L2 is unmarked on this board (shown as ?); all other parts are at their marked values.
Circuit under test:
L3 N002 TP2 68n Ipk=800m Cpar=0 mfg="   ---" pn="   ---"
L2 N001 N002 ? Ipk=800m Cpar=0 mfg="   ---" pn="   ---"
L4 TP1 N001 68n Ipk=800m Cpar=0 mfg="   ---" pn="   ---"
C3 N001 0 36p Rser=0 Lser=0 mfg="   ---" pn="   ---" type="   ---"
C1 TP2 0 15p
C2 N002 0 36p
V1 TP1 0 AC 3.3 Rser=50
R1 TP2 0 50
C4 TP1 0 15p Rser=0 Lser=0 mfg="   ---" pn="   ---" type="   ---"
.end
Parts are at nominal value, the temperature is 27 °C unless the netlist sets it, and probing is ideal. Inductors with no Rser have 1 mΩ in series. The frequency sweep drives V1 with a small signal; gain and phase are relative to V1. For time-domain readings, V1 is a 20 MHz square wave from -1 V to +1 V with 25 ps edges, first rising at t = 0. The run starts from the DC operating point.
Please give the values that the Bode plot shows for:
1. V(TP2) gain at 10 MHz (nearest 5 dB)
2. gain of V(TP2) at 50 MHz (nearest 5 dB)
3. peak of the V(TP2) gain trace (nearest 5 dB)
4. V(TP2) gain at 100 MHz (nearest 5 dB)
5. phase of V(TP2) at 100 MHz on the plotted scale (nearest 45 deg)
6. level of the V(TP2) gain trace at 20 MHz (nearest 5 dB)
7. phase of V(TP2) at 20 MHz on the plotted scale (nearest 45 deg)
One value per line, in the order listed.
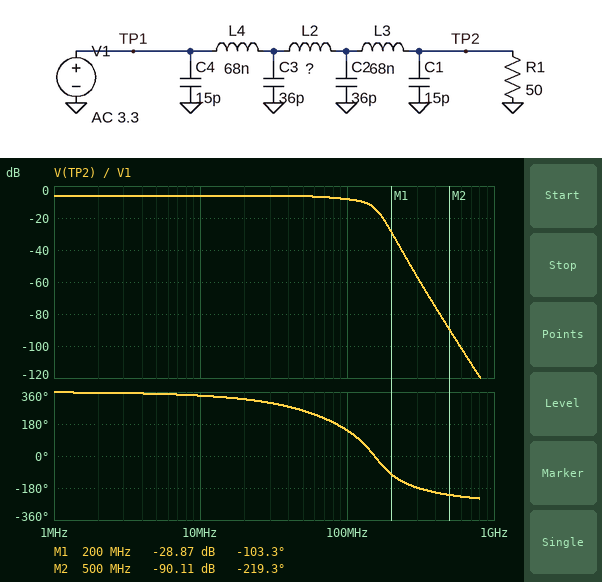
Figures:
-5 dB
-5 dB
-5 dB
-10 dB
135 deg
-5 dB
315 deg
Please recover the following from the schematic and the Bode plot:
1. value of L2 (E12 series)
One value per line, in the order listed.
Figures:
180 nH
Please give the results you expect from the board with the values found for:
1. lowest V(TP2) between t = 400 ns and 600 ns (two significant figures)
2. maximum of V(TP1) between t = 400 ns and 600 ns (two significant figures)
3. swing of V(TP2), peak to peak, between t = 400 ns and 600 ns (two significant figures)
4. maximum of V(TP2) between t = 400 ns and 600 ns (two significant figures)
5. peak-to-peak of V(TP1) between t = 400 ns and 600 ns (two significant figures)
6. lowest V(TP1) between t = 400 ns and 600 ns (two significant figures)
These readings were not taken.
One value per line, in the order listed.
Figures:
-580 mV
900 mV
1.2 V
580 mV
1.8 V
-900 mV
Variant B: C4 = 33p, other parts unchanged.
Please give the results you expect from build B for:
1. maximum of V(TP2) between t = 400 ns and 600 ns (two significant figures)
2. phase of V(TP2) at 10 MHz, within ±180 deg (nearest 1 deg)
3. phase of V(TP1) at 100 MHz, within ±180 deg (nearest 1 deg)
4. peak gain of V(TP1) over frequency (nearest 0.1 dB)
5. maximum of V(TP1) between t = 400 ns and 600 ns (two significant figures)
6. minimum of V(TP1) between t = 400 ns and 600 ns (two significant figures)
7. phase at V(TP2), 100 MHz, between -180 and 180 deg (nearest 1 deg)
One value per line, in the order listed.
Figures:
560 mV
-22 deg
-48 deg
-0.5 dB
840 mV
-840 mV
135 deg
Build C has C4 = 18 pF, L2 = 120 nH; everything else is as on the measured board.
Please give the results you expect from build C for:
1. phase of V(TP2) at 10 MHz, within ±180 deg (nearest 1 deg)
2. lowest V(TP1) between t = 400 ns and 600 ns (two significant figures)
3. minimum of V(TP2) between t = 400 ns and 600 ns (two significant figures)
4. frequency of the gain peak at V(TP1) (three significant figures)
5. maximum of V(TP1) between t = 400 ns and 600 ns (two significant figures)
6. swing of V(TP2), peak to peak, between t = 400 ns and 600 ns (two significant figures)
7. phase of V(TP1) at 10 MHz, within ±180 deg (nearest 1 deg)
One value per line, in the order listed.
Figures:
-19 deg
-730 mV
-650 mV
188 MHz
730 mV
1.3 V
0 deg
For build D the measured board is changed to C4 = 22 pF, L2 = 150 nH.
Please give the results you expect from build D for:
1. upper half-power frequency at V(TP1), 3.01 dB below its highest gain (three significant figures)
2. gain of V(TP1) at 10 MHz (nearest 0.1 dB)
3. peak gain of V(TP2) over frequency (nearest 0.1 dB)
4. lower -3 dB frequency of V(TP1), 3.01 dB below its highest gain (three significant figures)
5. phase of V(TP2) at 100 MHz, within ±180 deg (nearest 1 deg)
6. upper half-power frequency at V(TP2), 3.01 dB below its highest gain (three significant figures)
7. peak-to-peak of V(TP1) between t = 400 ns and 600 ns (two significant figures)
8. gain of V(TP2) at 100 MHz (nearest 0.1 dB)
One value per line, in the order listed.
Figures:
239 MHz
-6.0 dB
-6.0 dB
153 MHz
148 deg
144 MHz
1.6 V
-7.7 dB
